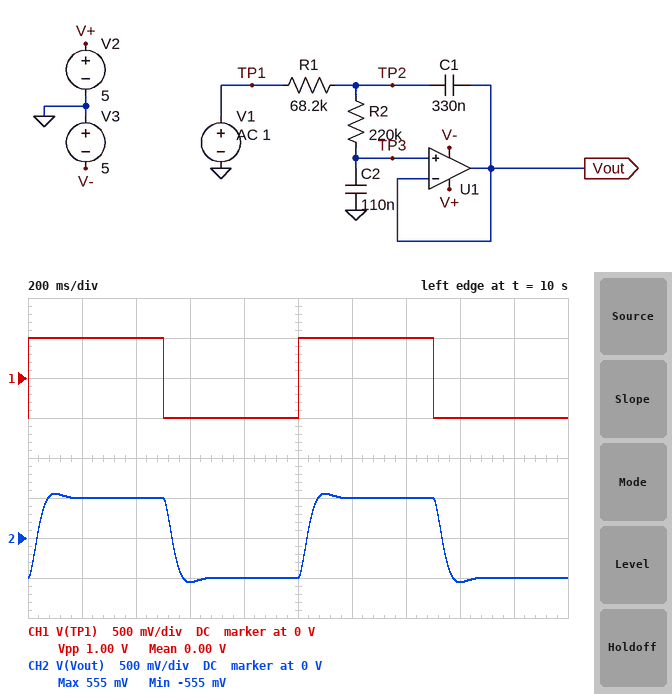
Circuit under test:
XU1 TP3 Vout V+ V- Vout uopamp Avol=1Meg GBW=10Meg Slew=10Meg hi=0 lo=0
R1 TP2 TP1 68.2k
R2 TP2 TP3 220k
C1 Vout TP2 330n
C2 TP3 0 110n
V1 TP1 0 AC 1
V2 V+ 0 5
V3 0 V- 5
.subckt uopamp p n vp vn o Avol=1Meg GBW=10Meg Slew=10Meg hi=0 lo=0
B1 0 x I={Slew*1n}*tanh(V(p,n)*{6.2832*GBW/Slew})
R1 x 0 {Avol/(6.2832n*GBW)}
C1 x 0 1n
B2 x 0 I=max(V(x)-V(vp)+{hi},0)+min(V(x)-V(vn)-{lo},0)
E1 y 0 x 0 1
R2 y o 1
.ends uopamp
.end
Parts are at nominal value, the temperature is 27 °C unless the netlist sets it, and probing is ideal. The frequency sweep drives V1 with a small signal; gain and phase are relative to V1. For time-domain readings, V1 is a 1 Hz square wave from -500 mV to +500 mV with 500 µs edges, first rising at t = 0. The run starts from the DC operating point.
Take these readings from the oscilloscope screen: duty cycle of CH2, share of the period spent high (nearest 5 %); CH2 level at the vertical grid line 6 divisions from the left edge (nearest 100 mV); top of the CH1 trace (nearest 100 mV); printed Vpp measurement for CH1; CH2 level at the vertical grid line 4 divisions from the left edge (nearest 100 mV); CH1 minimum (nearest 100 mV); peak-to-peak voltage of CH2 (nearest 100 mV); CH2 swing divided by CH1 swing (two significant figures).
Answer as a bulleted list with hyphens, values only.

- 50 %
- 500 mV
- 500 mV
- 1.00 V
- -500 mV
- -500 mV
- 1.1 V
- 1.1
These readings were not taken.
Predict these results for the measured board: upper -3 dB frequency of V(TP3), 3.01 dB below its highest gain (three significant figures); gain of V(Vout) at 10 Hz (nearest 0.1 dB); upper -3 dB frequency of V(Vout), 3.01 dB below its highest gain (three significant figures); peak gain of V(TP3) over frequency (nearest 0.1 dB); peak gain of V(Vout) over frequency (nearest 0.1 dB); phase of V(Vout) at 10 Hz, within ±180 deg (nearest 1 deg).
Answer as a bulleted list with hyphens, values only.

- 7.07 Hz
- -7.2 dB
- 7.07 Hz
- 0 dB
- 0 dB
- -120 deg
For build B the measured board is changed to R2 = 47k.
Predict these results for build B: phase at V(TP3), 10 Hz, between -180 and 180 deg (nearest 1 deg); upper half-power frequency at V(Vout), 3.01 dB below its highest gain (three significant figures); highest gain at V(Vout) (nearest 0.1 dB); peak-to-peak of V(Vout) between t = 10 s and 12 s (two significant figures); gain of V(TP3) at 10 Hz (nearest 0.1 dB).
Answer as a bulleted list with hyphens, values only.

- -56 deg
- 16.6 Hz
- 0.4 dB
- 1.2 V
- 0.3 dB
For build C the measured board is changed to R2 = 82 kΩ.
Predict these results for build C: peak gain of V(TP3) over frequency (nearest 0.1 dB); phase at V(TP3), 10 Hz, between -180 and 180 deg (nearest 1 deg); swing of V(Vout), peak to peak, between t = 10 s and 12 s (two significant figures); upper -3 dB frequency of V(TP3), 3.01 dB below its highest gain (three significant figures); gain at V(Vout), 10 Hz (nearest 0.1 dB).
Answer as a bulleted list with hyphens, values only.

- 0.5 dB
- -79 deg
- 1.2 V
- 12.6 Hz
- -0.5 dB
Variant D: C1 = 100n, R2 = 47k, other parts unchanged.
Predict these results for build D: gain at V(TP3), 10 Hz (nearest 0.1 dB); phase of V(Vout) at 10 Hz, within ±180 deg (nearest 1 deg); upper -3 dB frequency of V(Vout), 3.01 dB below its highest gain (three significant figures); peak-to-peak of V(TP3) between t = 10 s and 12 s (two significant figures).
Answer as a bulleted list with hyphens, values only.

- -1.4 dB
- -43 deg
- 15.7 Hz
- 1.0 V
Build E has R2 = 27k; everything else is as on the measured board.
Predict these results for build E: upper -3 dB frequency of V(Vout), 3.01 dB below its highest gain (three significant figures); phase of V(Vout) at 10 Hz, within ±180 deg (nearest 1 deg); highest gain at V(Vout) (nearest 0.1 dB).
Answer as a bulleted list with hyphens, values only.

- 21.0 Hz
- -42 deg
- 0.1 dB
